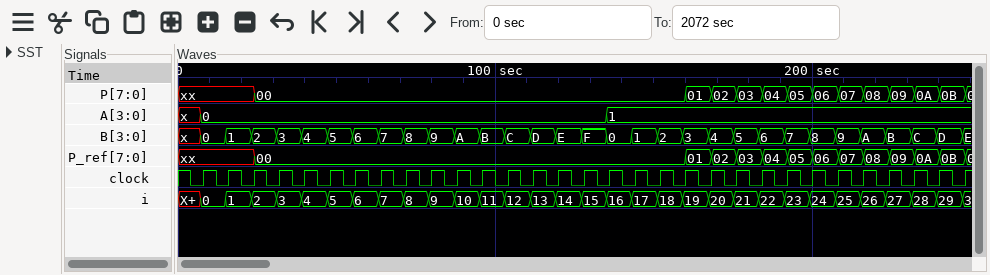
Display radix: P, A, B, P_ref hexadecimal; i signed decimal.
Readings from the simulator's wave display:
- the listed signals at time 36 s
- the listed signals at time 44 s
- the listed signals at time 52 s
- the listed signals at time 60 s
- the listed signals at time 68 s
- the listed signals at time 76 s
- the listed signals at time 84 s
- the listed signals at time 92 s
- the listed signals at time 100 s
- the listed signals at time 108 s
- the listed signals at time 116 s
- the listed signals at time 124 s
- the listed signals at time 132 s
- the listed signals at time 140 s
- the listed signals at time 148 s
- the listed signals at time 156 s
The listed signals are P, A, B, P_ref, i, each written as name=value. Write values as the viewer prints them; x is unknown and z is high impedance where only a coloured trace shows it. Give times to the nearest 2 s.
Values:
P=00, A=0, B=3, P_ref=00, i=3
P=00, A=0, B=4, P_ref=00, i=4
P=00, A=0, B=5, P_ref=00, i=5
P=00, A=0, B=6, P_ref=00, i=6
P=00, A=0, B=7, P_ref=00, i=7
P=00, A=0, B=8, P_ref=00, i=8
P=00, A=0, B=9, P_ref=00, i=9
P=00, A=0, B=A, P_ref=00, i=10
P=00, A=0, B=B, P_ref=00, i=11
P=00, A=0, B=C, P_ref=00, i=12
P=00, A=0, B=D, P_ref=00, i=13
P=00, A=0, B=E, P_ref=00, i=14
P=00, A=0, B=F, P_ref=00, i=15
P=00, A=1, B=0, P_ref=00, i=16
P=00, A=1, B=1, P_ref=00, i=17
P=00, A=1, B=2, P_ref=00, i=18
